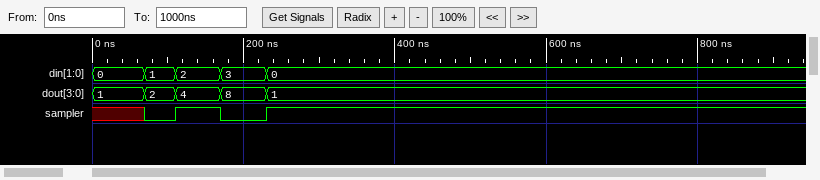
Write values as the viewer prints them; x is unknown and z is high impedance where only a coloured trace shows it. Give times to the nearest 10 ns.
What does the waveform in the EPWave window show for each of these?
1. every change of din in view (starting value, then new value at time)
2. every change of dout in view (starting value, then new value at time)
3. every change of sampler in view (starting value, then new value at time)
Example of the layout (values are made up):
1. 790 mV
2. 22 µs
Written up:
1. 0, 1 at 70 ns, 2 at 110 ns, 3 at 170 ns, 0 at 230 ns
2. 1, 2 at 70 ns, 4 at 110 ns, 8 at 170 ns, 1 at 230 ns
3. x, 0 at 70 ns, 1 at 110 ns, 0 at 170 ns, 1 at 230 ns
